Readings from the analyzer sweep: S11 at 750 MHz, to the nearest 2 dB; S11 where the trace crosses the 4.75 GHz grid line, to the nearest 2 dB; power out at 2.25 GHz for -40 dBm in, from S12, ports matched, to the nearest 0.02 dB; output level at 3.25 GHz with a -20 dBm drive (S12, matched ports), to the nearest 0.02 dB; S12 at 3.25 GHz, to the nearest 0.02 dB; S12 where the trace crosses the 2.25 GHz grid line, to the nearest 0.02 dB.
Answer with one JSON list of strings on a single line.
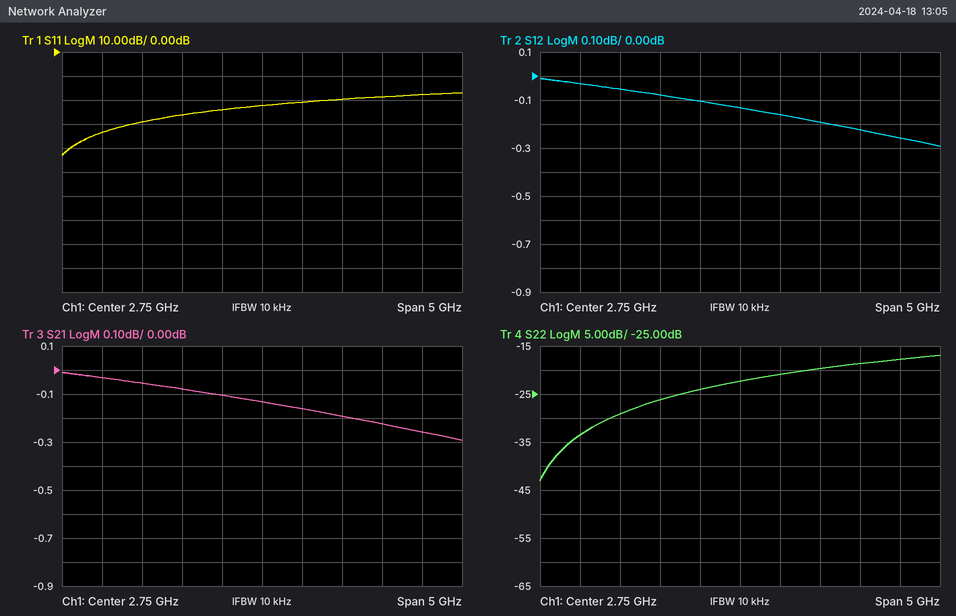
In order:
["-34 dB", "-18 dB", "-40.10 dBm", "-20.16 dBm", "-0.16 dB", "-0.10 dB"]
